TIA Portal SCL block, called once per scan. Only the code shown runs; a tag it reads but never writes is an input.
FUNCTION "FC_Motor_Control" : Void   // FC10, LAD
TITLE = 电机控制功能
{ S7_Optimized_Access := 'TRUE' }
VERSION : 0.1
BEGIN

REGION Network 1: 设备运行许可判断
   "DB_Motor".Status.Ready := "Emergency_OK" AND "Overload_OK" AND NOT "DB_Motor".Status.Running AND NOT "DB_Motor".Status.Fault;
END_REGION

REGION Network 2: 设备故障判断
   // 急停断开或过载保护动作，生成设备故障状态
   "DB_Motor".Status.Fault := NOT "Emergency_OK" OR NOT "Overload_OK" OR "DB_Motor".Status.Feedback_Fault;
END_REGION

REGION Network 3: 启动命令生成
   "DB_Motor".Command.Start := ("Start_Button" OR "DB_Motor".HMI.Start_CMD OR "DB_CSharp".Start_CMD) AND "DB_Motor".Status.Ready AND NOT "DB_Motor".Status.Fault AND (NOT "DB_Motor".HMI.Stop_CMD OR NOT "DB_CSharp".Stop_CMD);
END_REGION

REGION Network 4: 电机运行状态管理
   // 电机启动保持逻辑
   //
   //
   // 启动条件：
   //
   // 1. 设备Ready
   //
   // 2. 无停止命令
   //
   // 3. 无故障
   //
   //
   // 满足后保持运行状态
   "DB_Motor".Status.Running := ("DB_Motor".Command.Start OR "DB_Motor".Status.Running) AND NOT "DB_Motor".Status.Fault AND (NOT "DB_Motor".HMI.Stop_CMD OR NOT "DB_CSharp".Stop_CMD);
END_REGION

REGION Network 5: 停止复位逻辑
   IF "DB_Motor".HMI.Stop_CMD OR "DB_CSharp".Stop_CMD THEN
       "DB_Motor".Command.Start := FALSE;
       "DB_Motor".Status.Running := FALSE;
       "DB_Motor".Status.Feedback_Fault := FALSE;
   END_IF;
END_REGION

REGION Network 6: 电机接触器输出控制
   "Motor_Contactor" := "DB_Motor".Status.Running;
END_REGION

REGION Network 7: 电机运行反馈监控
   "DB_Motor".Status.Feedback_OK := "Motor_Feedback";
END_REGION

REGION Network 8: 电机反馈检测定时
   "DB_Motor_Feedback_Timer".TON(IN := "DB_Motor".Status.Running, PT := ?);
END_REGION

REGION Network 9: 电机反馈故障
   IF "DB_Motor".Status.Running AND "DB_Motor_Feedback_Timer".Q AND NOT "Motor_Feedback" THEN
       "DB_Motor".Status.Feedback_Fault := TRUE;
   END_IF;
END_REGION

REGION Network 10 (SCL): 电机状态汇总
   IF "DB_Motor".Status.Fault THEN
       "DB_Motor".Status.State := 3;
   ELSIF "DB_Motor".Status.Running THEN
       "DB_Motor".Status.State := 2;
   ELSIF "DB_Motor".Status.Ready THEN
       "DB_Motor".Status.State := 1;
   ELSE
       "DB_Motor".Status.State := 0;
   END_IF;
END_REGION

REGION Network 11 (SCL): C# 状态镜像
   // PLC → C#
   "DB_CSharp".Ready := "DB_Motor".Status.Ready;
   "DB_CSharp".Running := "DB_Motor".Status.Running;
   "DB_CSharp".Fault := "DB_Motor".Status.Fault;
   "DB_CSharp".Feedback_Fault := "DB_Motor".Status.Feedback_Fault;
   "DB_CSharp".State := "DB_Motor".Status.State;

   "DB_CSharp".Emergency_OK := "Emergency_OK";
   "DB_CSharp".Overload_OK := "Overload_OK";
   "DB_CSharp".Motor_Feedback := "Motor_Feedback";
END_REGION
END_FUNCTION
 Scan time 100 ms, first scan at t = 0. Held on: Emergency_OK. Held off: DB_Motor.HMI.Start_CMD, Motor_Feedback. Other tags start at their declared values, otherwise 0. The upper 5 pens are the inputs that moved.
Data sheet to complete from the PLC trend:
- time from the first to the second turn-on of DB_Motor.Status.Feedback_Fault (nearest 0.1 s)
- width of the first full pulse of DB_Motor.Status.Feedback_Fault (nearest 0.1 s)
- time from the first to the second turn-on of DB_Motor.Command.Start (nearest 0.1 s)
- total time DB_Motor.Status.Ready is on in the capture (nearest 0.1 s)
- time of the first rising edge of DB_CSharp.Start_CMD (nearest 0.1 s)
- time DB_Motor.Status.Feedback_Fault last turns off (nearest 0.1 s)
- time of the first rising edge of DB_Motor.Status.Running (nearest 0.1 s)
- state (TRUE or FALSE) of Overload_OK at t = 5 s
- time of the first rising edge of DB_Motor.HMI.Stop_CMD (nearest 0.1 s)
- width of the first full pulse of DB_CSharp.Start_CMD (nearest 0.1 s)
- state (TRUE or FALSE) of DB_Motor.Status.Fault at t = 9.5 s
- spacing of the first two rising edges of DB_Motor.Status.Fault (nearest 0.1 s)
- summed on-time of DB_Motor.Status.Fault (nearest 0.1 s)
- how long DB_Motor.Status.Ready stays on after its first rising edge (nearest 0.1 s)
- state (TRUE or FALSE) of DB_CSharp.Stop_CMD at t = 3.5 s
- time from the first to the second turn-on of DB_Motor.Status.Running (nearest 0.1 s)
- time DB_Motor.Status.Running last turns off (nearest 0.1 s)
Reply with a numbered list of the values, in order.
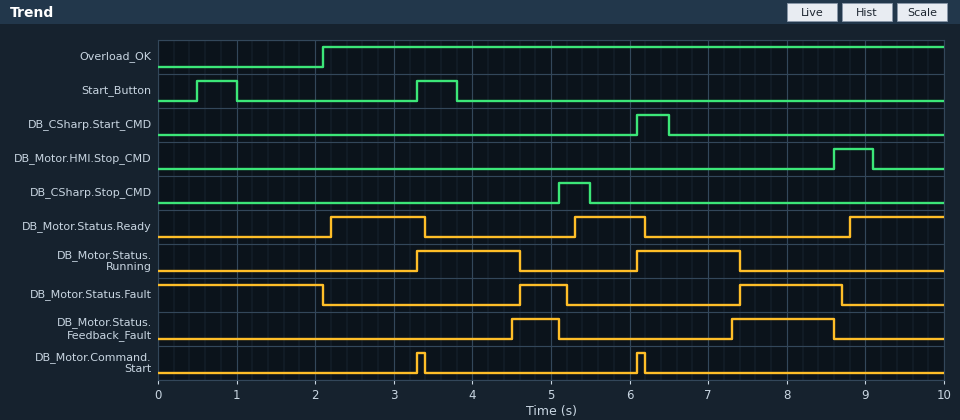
1. 2.8 s
2. 0.6 s
3. 2.8 s
4. 3.3 s
5. 6.1 s
6. 8.6 s
7. 3.3 s
8. TRUE
9. 8.6 s
10. 0.4 s
11. FALSE
12. 2.8 s
13. 4.0 s
14. 1.2 s
15. FALSE
16. 2.8 s
17. 7.4 s
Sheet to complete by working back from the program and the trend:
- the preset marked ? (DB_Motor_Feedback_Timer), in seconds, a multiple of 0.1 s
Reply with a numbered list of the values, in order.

1. 1.2 s
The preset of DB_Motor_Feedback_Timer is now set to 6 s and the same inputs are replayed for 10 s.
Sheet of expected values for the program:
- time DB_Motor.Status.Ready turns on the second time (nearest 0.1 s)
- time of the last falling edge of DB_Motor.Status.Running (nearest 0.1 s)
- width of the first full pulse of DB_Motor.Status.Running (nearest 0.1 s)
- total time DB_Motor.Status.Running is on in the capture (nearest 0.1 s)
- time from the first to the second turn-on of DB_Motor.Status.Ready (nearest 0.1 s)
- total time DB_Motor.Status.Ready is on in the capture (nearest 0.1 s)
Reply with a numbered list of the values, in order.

1. 5.2 s
2. 8.6 s
3. 1.8 s
4. 4.3 s
5. 3.0 s
6. 3.5 s
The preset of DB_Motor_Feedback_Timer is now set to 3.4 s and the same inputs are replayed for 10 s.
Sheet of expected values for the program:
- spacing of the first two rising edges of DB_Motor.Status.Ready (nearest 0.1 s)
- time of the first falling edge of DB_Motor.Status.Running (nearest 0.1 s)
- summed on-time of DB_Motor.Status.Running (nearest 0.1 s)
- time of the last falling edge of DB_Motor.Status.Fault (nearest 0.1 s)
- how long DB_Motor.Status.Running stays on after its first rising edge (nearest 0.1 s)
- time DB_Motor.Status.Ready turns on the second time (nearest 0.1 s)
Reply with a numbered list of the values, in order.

1. 3.0 s
2. 5.1 s
3. 4.3 s
4. 2.1 s
5. 1.8 s
6. 5.2 s
